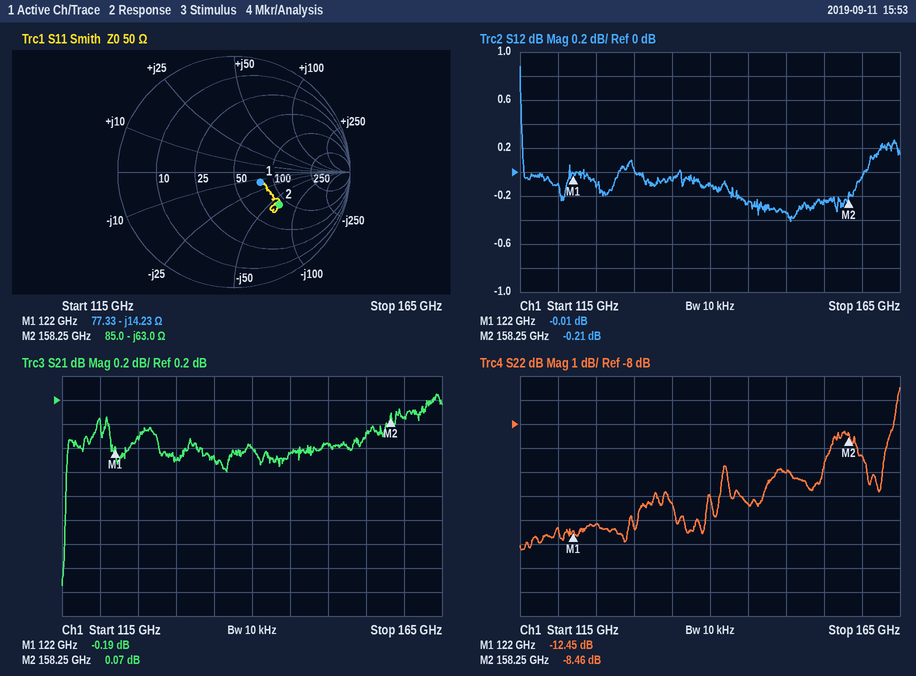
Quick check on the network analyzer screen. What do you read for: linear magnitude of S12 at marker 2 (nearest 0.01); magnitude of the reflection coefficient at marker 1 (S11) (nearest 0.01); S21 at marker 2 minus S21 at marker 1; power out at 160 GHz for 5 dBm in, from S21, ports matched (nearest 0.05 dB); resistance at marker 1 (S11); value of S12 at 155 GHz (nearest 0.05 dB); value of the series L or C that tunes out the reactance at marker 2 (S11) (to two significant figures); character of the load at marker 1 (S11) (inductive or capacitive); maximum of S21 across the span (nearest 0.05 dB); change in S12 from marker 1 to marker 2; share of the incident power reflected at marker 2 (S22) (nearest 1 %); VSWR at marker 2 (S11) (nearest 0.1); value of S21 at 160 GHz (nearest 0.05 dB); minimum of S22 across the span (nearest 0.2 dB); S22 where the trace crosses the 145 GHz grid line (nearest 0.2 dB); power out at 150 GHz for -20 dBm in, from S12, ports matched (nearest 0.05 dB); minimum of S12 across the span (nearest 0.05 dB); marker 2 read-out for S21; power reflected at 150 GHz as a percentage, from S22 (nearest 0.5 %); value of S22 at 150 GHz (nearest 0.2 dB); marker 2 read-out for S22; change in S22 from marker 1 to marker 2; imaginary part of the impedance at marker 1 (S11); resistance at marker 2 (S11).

0.98
0.24
0.26 dB
5.05 dBm
77.33 Ω
-0.25 dB
63 pH
capacitive
0.25 dB
-0.20 dB
14 %
2.9
0.05 dB
-13.2 dB
-11.4 dB
-20.35 dBm
-0.40 dB
0.07 dB
10.0 %
-10.0 dB
-8.46 dB
3.99 dB
-14.23 Ω
85.0 Ω
